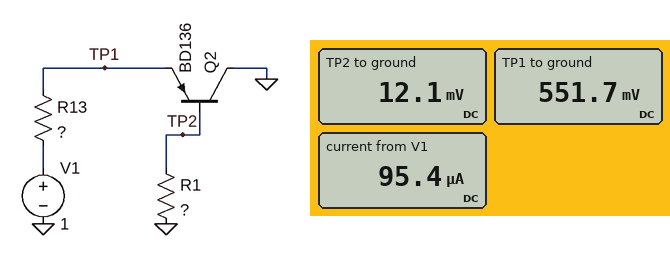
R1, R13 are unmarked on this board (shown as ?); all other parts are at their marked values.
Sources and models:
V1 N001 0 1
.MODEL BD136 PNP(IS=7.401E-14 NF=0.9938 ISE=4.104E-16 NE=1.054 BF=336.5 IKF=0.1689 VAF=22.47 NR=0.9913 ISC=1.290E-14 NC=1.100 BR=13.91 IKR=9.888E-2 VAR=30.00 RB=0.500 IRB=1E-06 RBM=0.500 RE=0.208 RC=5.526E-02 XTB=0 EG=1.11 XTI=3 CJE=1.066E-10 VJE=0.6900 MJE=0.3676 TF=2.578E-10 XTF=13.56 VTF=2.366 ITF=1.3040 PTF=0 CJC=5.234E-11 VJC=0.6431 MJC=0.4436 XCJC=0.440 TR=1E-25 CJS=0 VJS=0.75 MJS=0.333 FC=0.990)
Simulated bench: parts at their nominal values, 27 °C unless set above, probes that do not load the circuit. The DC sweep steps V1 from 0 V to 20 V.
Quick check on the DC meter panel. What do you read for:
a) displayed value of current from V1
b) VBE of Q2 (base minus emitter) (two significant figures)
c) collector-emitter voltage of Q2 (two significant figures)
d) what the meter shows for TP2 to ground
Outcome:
95.4 µA
-540 mV
-550 mV
12.1 mV
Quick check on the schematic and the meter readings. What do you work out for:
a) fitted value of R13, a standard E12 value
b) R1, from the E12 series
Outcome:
4.7 kΩ
27 kΩ
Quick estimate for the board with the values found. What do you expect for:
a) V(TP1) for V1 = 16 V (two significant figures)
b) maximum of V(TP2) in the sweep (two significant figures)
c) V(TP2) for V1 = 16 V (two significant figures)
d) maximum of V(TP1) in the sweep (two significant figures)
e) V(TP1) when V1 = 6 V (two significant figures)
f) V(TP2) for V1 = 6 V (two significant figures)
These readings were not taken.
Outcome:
1.0 V
480 mV
380 mV
1.1 V
740 mV
140 mV
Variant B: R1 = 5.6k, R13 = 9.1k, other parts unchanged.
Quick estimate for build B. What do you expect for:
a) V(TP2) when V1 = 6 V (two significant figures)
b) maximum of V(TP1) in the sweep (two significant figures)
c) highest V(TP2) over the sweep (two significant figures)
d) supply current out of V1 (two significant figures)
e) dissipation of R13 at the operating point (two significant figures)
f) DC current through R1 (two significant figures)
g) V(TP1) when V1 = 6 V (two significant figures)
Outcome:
15 mV
670 mV
53 mV
52 µA
25 µW
250 nA
600 mV
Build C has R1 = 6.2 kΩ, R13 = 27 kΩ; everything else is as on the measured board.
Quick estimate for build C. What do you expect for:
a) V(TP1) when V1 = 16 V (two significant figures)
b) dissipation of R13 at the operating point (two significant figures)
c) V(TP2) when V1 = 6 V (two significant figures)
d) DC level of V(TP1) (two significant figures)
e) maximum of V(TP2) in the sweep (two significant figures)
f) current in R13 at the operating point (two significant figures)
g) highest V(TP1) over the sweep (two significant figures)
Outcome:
600 mV
9.3 µW
5.8 mV
500 mV
20 mV
19 µA
610 mV
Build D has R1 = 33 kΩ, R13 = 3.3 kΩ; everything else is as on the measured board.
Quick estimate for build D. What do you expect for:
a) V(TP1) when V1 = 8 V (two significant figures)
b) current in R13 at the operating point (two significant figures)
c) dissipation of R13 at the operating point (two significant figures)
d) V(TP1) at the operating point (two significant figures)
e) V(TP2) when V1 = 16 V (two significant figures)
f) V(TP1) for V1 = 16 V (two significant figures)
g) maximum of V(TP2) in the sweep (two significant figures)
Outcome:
930 mV
130 µA
57 µW
570 mV
640 mV
1.3 V
810 mV
